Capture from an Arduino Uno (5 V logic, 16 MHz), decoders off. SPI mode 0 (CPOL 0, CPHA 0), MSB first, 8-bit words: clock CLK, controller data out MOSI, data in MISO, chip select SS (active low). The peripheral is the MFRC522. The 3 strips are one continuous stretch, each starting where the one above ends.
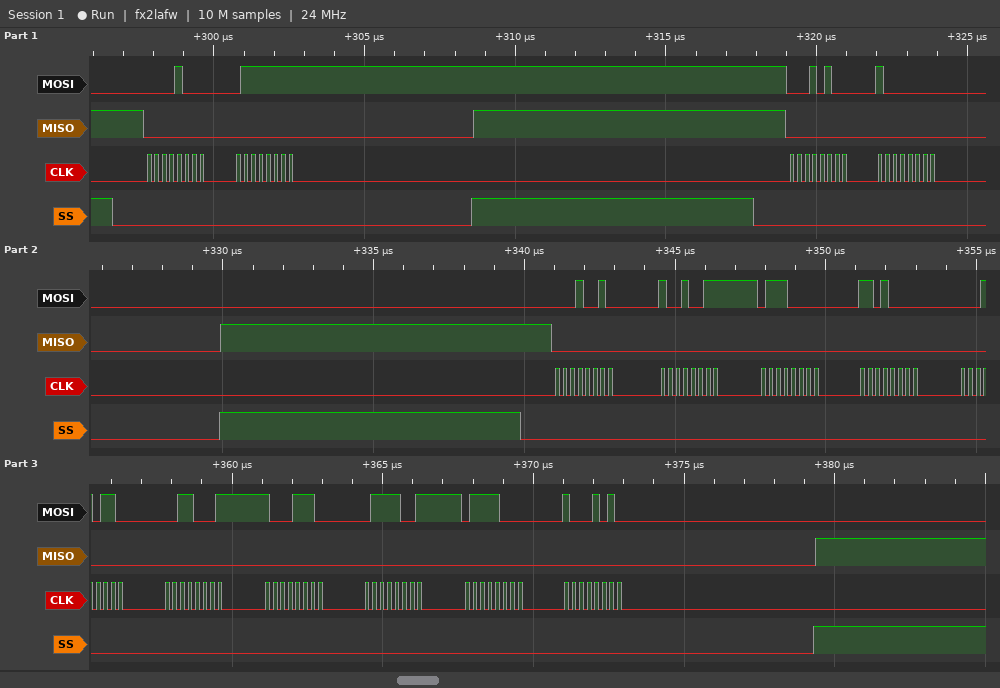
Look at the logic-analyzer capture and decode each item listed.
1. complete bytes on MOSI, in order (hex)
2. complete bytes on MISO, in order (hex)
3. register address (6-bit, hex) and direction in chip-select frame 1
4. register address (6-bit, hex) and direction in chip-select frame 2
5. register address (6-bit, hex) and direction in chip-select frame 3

08 7F 14 80 12 93 70 D0 16 31 8E 79 78 8A
00 00 00 00 00 00 00 00 00 00 00 00 00 00
0x04 write
0x0A write
0x09 write
